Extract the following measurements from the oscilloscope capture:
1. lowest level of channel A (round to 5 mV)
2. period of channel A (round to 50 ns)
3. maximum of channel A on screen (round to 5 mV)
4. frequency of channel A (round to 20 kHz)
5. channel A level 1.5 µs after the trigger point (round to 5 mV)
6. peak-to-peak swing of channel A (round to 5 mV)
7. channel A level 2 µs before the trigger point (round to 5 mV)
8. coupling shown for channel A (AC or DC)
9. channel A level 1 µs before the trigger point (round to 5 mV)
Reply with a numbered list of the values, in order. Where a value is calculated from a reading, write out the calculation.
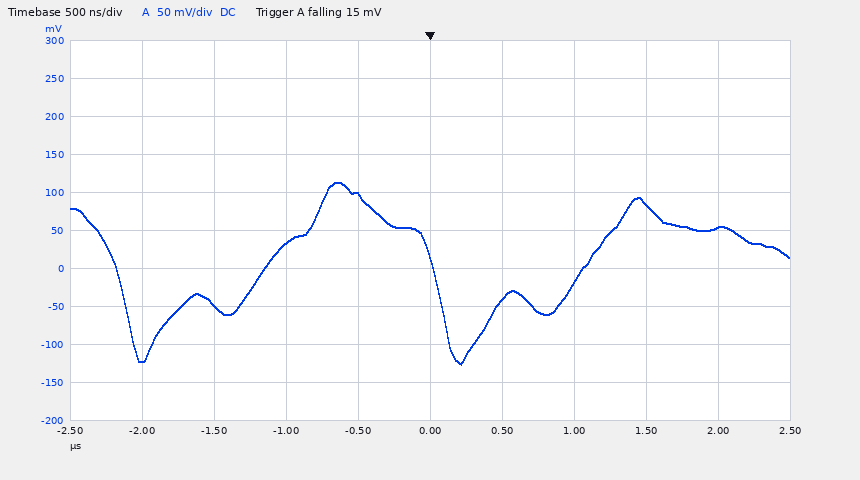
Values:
1. -125 mV
2. 2.20 µs
3. 115 mV
4. 1 / 2.20 µs ≈ 455 kHz, so 460 kHz to the nearest 20 kHz
5. 85 mV
6. 115 mV − (-125 mV) = 240 mV
7. -120 mV
8. DC
9. 35 mV
